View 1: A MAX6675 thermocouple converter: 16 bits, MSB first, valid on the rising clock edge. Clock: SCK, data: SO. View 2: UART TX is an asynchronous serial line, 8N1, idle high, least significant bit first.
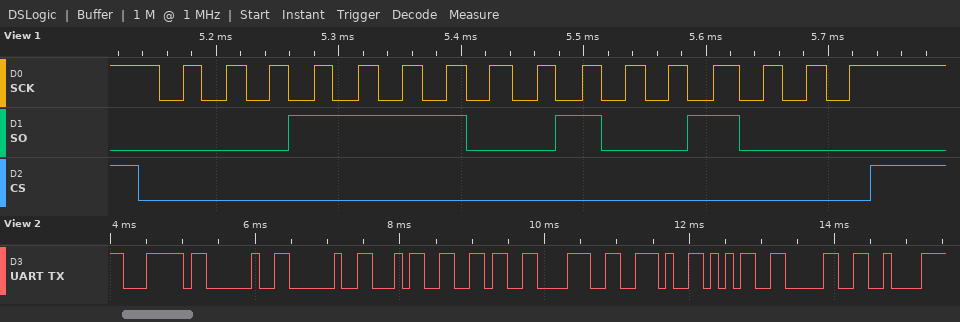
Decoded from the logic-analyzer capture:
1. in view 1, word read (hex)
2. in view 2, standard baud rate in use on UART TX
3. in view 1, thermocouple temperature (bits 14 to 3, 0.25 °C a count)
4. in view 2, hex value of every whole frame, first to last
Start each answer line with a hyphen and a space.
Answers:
- 0x1E48
- 9600 baud
- 242.25 °C
- 0x7C 0x20 0x20 0x34 0x36 0x38 0x2E 0x35 0x30 0xC2
